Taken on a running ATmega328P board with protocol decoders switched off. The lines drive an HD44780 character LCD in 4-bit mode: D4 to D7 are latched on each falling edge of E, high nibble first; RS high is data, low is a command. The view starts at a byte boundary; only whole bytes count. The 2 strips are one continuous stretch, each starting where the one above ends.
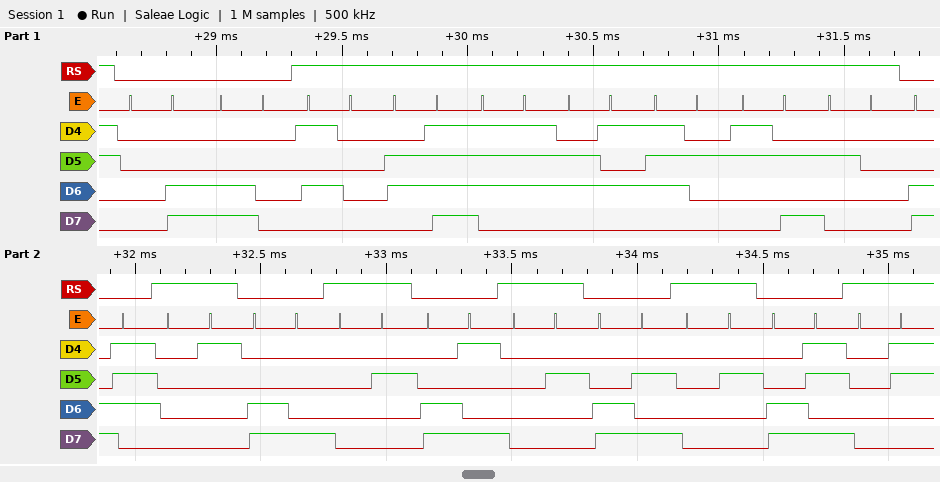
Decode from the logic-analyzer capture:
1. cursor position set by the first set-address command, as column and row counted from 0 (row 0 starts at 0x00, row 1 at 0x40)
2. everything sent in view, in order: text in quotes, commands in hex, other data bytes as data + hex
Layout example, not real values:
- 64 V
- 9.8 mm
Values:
- column 0, row 1
- 0x0C 0xC0 "Power: " 0xC7 data 01 0xC8 data 02 0xC9 data 02 0xCA data 02 0xCB data 03
